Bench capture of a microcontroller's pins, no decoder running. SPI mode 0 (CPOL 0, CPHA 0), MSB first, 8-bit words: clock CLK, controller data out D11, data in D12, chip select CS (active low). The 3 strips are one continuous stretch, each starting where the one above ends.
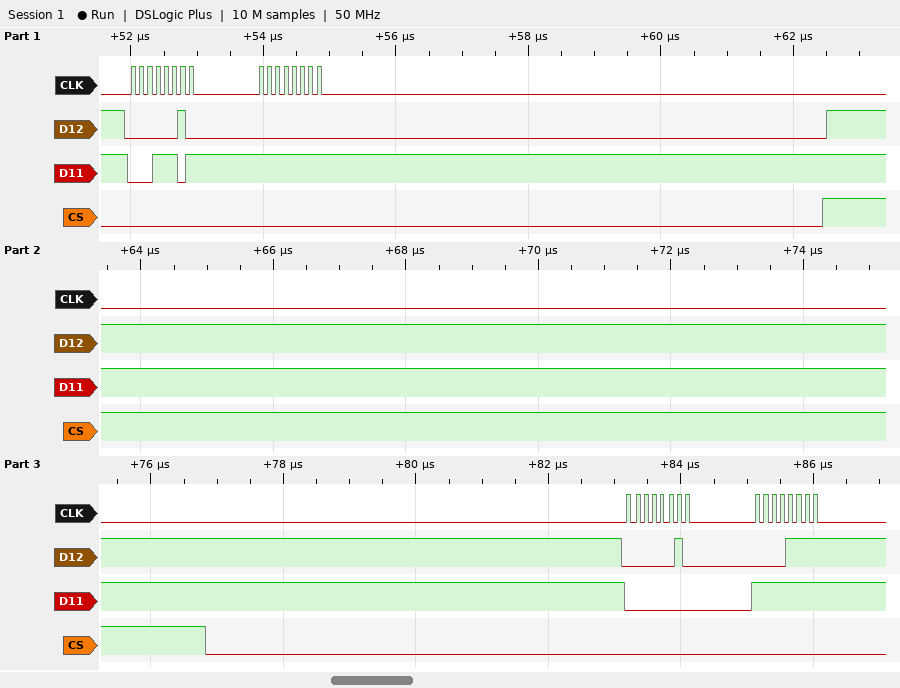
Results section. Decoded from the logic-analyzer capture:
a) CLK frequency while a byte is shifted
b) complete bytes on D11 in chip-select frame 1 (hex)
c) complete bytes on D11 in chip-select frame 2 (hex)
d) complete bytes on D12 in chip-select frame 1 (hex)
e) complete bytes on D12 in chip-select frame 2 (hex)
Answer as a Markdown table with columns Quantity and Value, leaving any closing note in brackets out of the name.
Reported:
| Quantity | Value |
|---|---|
| CLK frequency while a byte is shifted | 8 MHz |
| complete bytes on D11 in chip-select frame 1 | 0x1D 0xFF |
| complete bytes on D11 in chip-select frame 2 | 0x00 0xFF |
| complete bytes on D12 in chip-select frame 1 | 0x02 0x00 |
| complete bytes on D12 in chip-select frame 2 | 0x02 0x0F |
